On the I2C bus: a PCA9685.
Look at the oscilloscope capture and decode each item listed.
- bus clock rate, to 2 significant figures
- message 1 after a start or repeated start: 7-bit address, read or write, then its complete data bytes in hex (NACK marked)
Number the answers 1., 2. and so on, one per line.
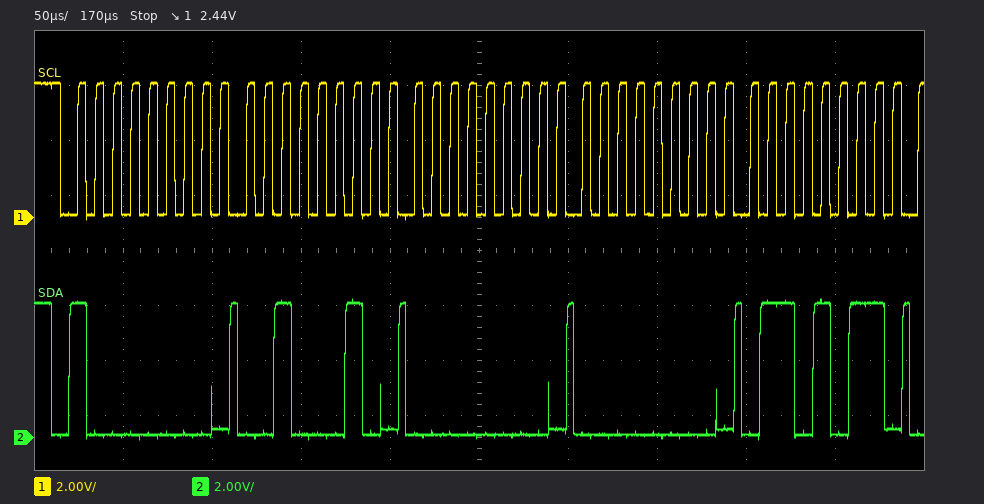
1. 100 kHz
2. 0x40 write: 22 00 00 6B
